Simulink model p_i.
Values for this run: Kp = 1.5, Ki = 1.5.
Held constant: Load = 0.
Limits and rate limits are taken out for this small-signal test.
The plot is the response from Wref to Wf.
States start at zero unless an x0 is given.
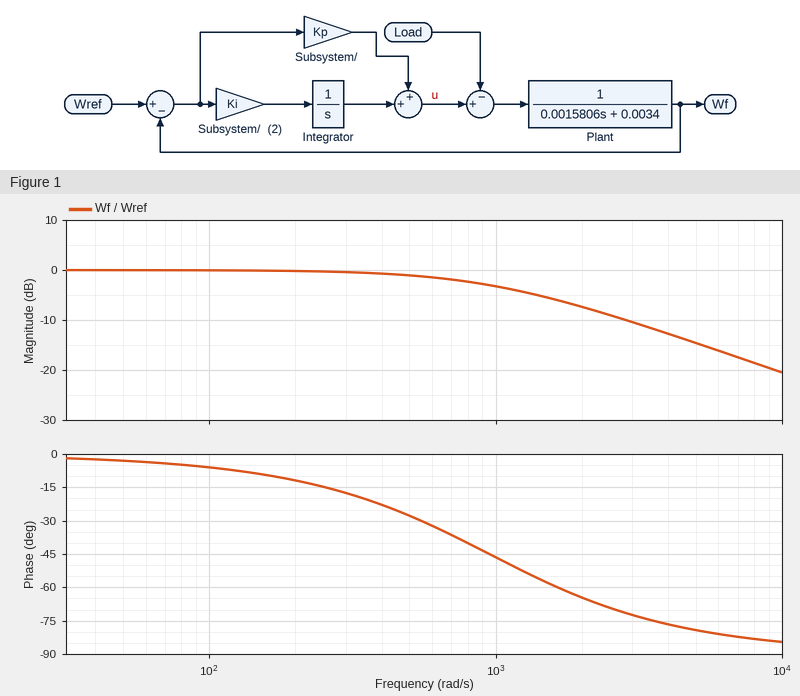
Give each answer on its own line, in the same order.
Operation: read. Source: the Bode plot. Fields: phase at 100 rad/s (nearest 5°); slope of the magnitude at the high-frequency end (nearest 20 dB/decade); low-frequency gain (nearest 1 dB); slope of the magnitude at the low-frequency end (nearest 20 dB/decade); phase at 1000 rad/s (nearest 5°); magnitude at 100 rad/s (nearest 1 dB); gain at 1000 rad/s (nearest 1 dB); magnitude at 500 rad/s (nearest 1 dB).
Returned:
-5°
-20 dB/decade
0 dB
0 dB/decade
-45°
0 dB
-3 dB
-1 dB
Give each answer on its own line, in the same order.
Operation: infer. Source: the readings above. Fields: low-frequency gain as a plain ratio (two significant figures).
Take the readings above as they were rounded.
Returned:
1.0
